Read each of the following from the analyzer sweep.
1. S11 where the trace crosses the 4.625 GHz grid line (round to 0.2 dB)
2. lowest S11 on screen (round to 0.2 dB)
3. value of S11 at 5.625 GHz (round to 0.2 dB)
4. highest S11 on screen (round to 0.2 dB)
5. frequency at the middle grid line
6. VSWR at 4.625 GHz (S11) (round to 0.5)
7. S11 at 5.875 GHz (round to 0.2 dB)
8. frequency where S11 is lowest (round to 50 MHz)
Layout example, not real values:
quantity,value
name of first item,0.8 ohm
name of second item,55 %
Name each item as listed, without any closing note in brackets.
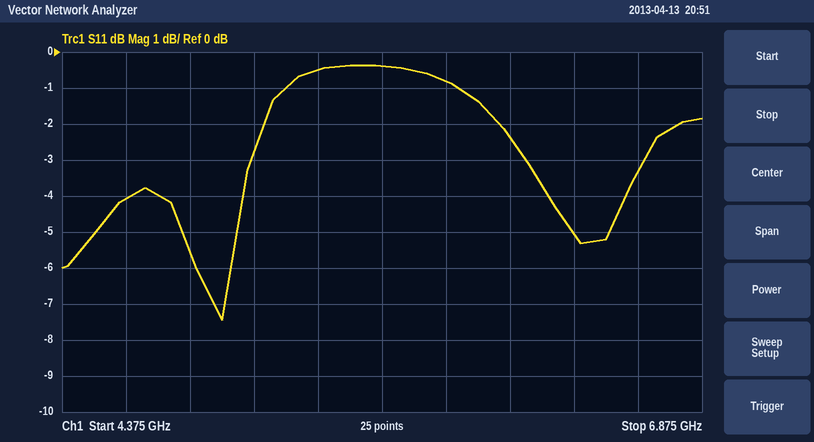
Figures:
quantity,value
S11 where the trace crosses the 4.625 GHz grid line,-4.0 dB
lowest S11 on screen,-7.4 dB
value of S11 at 5.625 GHz,-0.4 dB
highest S11 on screen,-0.4 dB
frequency at the middle grid line,5.625 GHz
VSWR at 4.625 GHz (S11),4.5
S11 at 5.875 GHz,-0.8 dB
frequency where S11 is lowest,5.00 GHz
